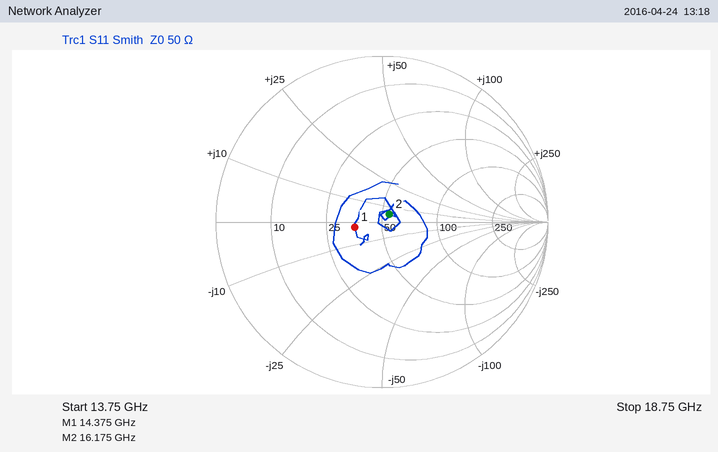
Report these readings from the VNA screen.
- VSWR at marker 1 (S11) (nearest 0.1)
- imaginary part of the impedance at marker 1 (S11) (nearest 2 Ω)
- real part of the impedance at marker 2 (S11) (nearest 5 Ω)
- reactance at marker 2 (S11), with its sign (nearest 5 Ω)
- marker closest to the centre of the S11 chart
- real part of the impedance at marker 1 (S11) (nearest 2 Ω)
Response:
1.4
-2 Ω
55 Ω
+5 Ω
marker 2
36 Ω
